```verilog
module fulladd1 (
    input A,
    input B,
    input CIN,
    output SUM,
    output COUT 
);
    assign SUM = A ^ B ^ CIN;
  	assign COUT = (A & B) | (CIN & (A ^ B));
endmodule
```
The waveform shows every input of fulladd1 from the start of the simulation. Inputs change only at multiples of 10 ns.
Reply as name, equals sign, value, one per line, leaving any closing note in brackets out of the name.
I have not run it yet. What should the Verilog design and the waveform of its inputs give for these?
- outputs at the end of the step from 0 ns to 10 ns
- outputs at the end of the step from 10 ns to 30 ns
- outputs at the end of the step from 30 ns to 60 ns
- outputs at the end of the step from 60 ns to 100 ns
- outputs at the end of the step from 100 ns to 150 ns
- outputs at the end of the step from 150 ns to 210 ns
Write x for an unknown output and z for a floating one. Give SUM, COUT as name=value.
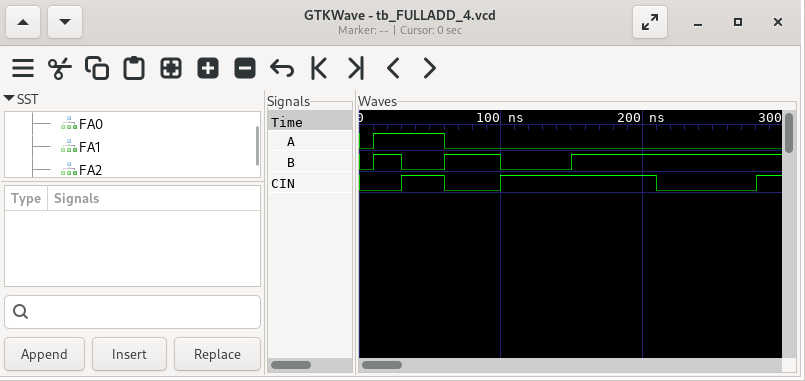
outputs at the end of the step from 0 ns to 10 ns = SUM=0, COUT=0
outputs at the end of the step from 10 ns to 30 ns = SUM=0, COUT=1
outputs at the end of the step from 30 ns to 60 ns = SUM=0, COUT=1
outputs at the end of the step from 60 ns to 100 ns = SUM=1, COUT=0
outputs at the end of the step from 100 ns to 150 ns = SUM=1, COUT=0
outputs at the end of the step from 150 ns to 210 ns = SUM=0, COUT=1
